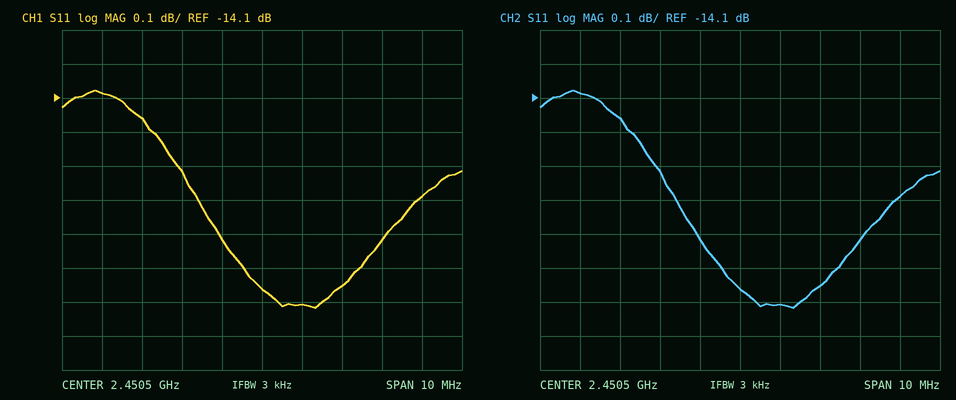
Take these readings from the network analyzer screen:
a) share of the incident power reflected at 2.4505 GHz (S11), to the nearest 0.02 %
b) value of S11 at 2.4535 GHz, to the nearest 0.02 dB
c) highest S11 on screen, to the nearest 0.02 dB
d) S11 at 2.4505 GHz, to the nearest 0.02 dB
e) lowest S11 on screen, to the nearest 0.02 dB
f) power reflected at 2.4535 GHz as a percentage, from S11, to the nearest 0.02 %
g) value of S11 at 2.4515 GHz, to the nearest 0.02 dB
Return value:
3.42 %
-14.52 dB
-14.08 dB
-14.66 dB
-14.72 dB
3.54 %
-14.70 dB
